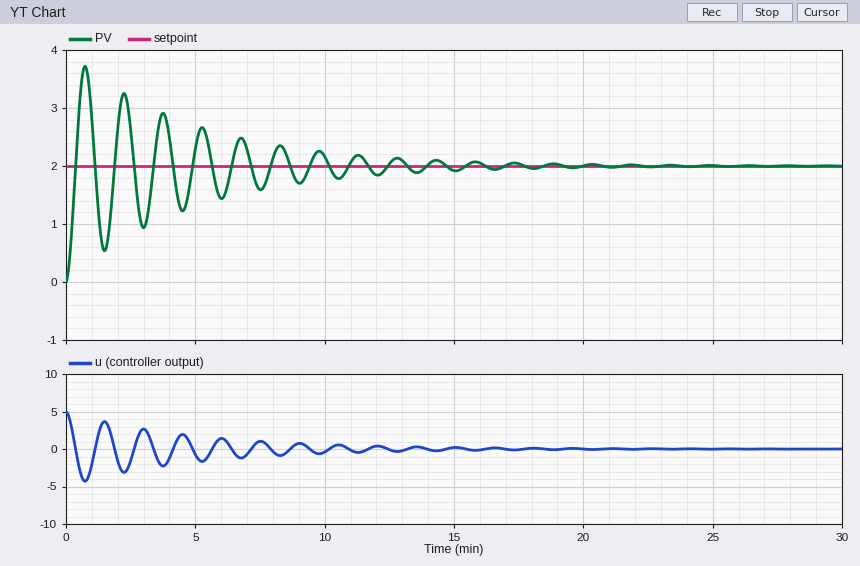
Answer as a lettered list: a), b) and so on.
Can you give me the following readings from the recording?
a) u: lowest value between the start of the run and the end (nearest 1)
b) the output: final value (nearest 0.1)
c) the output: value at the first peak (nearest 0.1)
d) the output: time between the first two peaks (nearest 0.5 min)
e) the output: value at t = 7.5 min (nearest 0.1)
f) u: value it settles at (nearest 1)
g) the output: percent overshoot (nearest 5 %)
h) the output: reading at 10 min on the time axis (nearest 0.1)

a) -4
b) 2.0
c) 3.7
d) 1.5 min
e) 1.6
f) 0
g) 85 %
h) 2.2
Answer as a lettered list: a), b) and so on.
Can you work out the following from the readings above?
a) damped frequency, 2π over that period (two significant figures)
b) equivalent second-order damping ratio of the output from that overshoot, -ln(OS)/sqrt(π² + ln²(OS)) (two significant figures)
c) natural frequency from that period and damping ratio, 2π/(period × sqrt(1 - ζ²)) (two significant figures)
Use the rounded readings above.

a) 4.2 rad/min
b) 0.052
c) 4.2 rad/min
